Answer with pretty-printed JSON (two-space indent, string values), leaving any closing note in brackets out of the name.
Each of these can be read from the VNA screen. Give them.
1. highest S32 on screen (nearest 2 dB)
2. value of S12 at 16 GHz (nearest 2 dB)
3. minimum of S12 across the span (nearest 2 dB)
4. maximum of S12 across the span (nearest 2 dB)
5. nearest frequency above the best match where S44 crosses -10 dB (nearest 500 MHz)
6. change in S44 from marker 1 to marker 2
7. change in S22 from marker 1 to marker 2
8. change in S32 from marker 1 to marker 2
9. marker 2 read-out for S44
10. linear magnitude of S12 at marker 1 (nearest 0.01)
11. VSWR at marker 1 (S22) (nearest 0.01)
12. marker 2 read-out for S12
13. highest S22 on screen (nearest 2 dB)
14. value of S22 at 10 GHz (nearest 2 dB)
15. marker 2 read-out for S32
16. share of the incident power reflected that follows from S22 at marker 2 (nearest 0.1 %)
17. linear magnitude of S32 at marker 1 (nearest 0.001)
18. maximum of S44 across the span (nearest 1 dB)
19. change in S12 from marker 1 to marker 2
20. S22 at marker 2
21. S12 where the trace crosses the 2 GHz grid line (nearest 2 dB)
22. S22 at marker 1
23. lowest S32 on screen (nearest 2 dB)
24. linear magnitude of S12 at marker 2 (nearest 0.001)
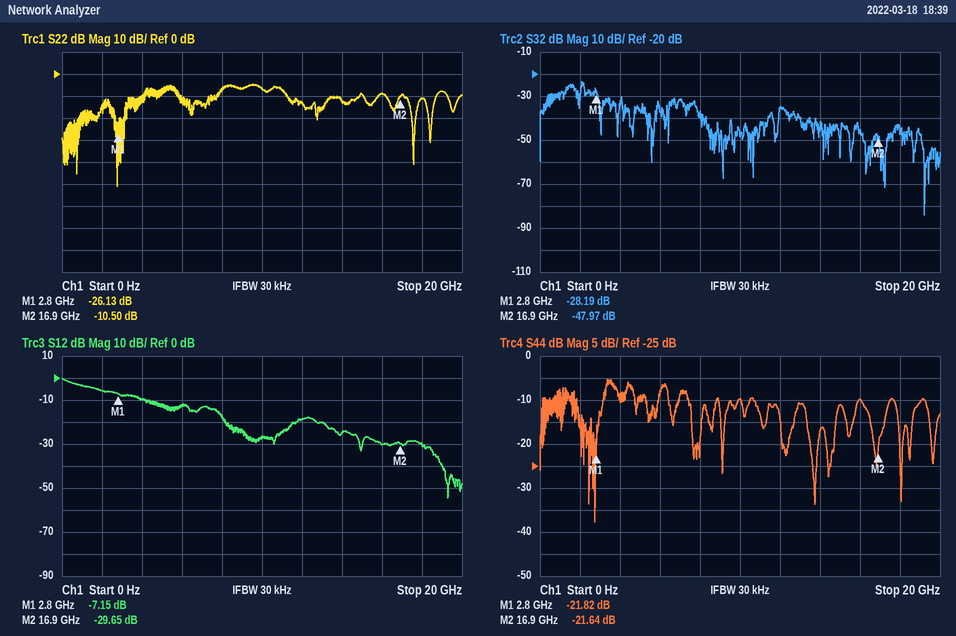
{
  "highest S32 on screen": "-24 dB",
  "value of S12 at 16 GHz": "-30 dB",
  "minimum of S12 across the span": "-54 dB",
  "maximum of S12 across the span": "0 dB",
  "nearest frequency above the best match where S44 crosses -10 dB": "3.0 GHz",
  "change in S44 from marker 1 to marker 2": "0.18 dB",
  "change in S22 from marker 1 to marker 2": "15.63 dB",
  "change in S32 from marker 1 to marker 2": "-19.78 dB",
  "marker 2 read-out for S44": "-21.64 dB",
  "linear magnitude of S12 at marker 1": "0.44",
  "VSWR at marker 1 (S22)": "1.10",
  "marker 2 read-out for S12": "-29.65 dB",
  "highest S22 on screen": "-4 dB",
  "value of S22 at 10 GHz": "-6 dB",
  "marker 2 read-out for S32": "-47.97 dB",
  "share of the incident power reflected that follows from S22 at marker 2": "8.9 %",
  "linear magnitude of S32 at marker 1": "0.039",
  "maximum of S44 across the span": "-5 dB",
  "change in S12 from marker 1 to marker 2": "-22.50 dB",
  "S22 at marker 2": "-10.50 dB",
  "S12 where the trace crosses the 2 GHz grid line": "-6 dB",
  "S22 at marker 1": "-26.13 dB",
  "lowest S32 on screen": "-84 dB",
  "linear magnitude of S12 at marker 2": "0.033"
}
